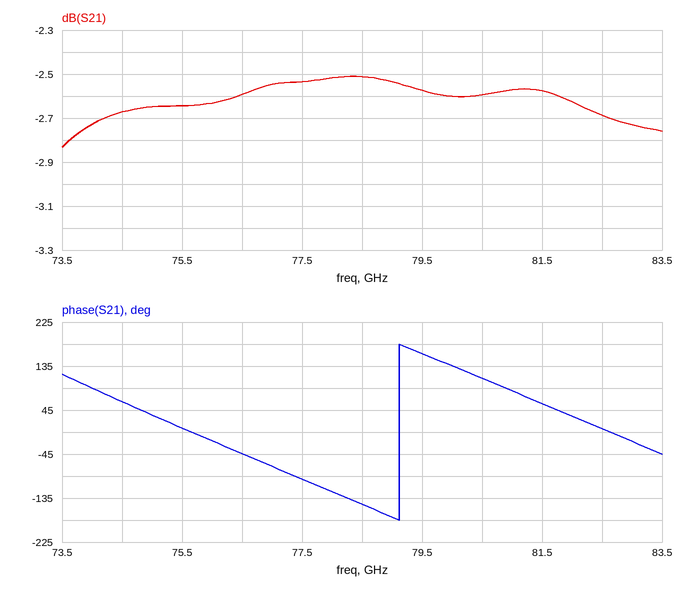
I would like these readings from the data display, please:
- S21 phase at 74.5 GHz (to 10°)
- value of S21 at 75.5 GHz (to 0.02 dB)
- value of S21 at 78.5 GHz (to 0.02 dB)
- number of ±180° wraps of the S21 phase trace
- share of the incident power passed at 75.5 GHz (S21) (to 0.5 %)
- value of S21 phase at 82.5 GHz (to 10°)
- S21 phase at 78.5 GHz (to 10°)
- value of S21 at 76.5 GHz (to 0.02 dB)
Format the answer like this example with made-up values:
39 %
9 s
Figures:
60°
-2.64 dB
-2.52 dB
1
54.5 %
10°
-150°
-2.60 dB
